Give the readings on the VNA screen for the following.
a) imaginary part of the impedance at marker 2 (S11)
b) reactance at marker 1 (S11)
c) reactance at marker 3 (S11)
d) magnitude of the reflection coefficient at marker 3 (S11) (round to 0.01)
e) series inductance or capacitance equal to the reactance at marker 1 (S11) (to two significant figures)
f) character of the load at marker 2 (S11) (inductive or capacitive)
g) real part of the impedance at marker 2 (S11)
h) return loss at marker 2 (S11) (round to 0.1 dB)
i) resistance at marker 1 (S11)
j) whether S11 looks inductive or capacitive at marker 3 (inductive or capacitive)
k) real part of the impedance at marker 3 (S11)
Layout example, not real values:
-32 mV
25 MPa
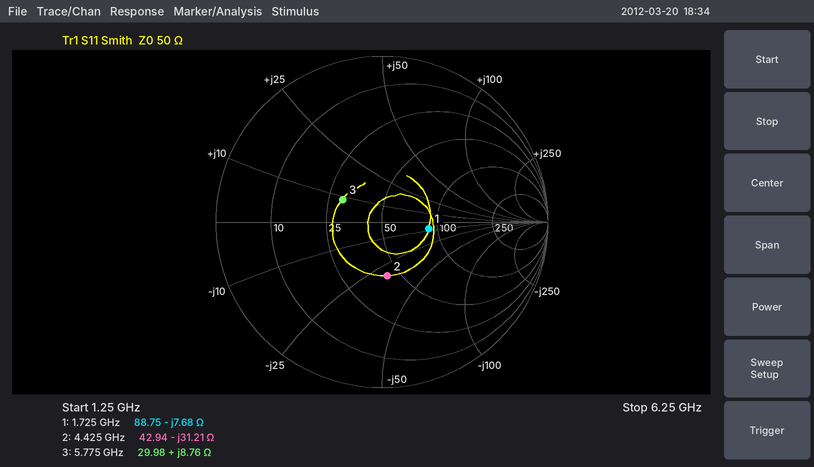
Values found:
-31.21 Ω
-7.68 Ω
+8.76 Ω
0.27
12 pF
capacitive
42.94 Ω
9.7 dB
88.75 Ω
inductive
29.98 Ω
